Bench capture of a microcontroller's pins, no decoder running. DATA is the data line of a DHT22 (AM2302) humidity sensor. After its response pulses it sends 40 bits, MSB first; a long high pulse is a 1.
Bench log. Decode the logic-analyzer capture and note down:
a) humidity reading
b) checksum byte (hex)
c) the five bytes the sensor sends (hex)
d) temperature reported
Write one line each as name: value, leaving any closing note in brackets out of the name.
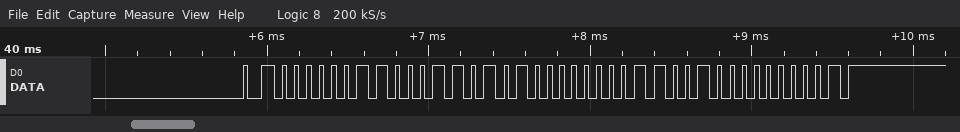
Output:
humidity reading: 79.4 %
checksum byte: 0x01
the five bytes the sensor sends: 03 1A 80 64 01
temperature reported: -10.0 °C
